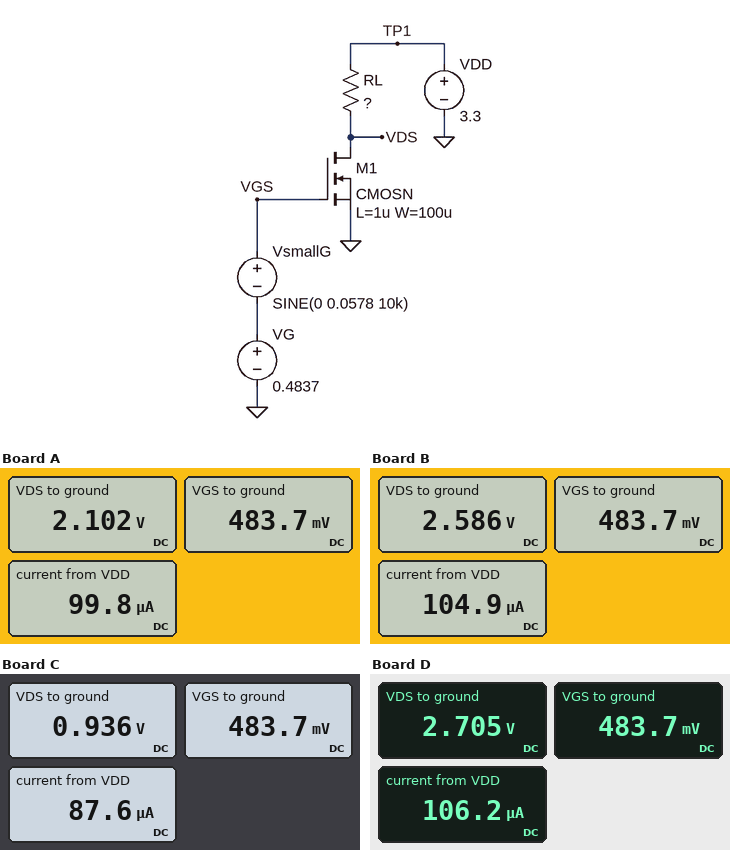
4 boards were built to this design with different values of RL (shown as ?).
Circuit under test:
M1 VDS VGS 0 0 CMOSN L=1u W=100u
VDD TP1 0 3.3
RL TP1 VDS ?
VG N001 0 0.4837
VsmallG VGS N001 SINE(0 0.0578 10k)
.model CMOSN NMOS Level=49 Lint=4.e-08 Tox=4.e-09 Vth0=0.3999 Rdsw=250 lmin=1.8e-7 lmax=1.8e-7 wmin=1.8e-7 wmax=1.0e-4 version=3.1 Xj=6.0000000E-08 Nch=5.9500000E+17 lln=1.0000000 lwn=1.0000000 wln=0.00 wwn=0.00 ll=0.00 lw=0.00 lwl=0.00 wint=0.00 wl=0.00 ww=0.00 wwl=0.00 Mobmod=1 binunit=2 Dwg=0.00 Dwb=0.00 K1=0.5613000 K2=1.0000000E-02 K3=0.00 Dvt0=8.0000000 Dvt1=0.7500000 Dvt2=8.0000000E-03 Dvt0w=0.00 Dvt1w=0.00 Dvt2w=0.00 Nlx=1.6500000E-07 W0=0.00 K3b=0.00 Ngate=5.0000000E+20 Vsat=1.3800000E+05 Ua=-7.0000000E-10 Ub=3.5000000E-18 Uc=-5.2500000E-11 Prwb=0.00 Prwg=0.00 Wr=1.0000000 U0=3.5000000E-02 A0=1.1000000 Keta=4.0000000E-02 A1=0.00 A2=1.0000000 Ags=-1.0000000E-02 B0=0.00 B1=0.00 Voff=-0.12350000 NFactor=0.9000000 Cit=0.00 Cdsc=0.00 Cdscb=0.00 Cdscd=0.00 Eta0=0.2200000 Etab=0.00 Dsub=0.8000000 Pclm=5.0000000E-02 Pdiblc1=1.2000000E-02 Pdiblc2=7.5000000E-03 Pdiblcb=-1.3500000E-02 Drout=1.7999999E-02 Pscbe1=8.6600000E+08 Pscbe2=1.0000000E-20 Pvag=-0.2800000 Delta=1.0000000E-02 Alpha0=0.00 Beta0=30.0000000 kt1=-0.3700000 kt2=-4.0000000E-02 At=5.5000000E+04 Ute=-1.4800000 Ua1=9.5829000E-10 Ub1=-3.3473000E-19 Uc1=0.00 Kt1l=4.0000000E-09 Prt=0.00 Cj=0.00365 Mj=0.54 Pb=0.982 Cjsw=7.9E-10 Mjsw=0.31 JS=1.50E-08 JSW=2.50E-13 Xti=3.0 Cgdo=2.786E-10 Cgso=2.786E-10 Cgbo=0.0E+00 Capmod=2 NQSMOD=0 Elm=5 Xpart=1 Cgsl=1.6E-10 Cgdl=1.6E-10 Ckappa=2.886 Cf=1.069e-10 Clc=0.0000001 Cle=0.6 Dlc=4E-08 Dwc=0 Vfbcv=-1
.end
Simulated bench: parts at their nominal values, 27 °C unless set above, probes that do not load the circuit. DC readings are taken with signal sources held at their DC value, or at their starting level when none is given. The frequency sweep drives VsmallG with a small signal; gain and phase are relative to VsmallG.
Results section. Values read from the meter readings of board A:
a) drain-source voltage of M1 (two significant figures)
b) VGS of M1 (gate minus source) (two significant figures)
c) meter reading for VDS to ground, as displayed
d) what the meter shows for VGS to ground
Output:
2.1 V
480 mV
2.102 V
483.7 mV
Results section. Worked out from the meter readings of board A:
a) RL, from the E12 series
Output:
12 kΩ
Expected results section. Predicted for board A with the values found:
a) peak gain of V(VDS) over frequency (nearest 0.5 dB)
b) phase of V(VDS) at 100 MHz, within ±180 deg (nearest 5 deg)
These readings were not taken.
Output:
25.0 dB
145 deg
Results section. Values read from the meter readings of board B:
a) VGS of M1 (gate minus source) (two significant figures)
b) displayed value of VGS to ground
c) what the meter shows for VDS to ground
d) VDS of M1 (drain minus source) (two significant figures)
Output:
480 mV
483.7 mV
2.586 V
2.6 V
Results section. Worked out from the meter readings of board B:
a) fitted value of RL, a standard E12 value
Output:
6.8 kΩ
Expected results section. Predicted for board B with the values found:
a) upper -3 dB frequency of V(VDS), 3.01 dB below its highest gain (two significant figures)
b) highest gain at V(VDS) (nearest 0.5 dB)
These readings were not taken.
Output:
250 MHz
21.0 dB
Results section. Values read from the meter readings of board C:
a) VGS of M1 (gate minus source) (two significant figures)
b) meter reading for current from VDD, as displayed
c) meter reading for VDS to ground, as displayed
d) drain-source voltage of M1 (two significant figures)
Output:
480 mV
87.6 µA
0.936 V
940 mV
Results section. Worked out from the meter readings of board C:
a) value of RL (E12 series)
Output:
27 kΩ
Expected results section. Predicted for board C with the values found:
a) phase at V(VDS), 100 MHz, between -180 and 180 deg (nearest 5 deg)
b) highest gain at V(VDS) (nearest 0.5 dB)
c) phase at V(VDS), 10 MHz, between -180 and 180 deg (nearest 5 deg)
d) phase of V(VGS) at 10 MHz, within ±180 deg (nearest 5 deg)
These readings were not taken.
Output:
120 deg
30.0 dB
170 deg
0 deg
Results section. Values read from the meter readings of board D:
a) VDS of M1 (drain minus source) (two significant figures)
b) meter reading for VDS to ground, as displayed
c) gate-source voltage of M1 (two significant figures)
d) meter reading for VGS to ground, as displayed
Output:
2.7 V
2.705 V
480 mV
483.7 mV
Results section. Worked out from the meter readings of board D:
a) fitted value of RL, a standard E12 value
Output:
5.6 kΩ
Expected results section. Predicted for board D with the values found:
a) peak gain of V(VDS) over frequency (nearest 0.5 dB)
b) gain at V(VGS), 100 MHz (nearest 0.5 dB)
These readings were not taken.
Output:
19.5 dB
0 dB
